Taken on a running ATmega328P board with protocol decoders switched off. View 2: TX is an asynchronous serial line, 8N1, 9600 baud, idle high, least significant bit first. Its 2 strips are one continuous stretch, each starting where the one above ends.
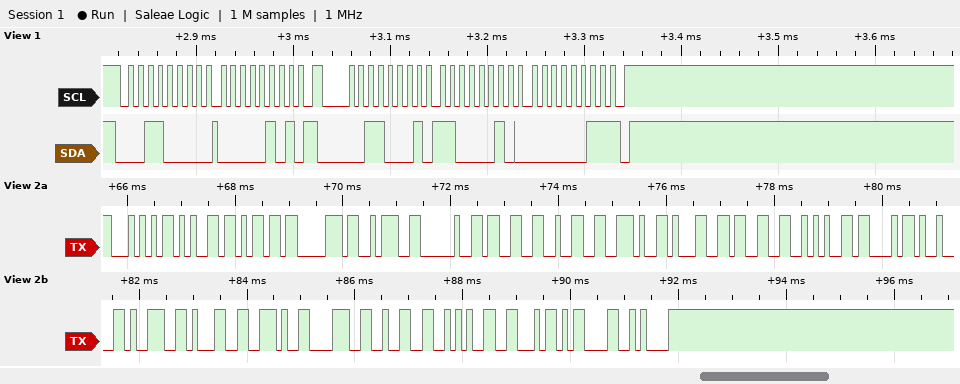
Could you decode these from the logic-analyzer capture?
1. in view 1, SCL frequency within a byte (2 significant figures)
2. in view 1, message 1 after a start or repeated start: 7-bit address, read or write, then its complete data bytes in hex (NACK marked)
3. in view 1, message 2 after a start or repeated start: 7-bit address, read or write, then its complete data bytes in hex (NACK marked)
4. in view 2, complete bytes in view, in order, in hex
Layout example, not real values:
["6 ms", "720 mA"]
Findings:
["100 kHz", "0x18 write: 05", "0x18 read: C2 03 NACK", "54 65 6D 70 3A 20 33 32 2E 31 33 2A 43 09 39 31 2E 38 32 2A 46 0D 0A"]
